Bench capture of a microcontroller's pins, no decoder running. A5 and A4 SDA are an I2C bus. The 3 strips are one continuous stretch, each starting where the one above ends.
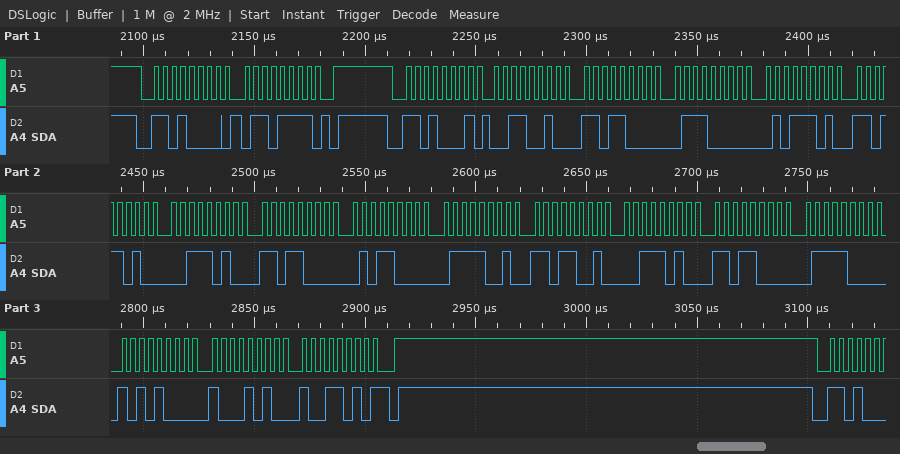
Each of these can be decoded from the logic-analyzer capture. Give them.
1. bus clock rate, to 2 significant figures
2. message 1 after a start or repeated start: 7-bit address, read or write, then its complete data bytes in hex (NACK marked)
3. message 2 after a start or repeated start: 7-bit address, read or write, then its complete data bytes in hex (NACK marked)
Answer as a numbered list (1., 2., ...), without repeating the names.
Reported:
1. 250 kHz
2. 0x68 write: 6F
3. 0x68 read: 32 D8 70 5D DA 3A D8 58 79 D9 3A D8 78 A8 8A 9A NACK
